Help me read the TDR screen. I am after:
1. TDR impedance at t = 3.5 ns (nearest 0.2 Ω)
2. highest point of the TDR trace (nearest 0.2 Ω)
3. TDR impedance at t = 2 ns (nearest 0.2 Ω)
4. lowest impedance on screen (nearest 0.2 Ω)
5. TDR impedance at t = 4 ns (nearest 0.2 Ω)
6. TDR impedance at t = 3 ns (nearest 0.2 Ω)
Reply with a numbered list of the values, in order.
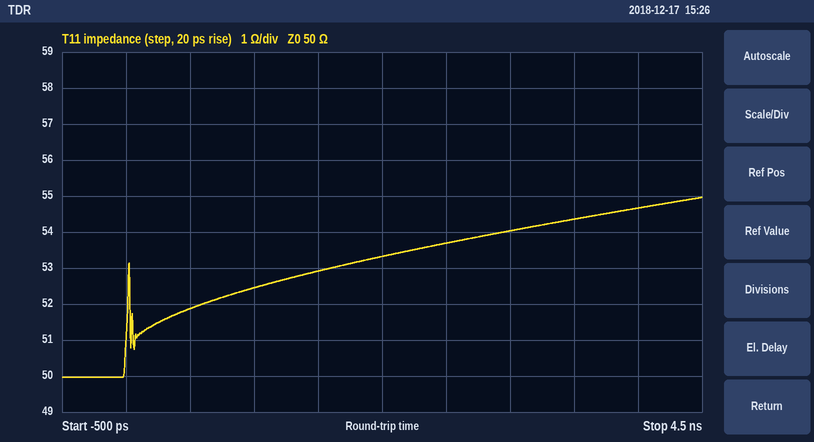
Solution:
1. 54.4 Ω
2. 55.0 Ω
3. 53.4 Ω
4. 50.0 Ω
5. 54.6 Ω
6. 54.0 Ω
